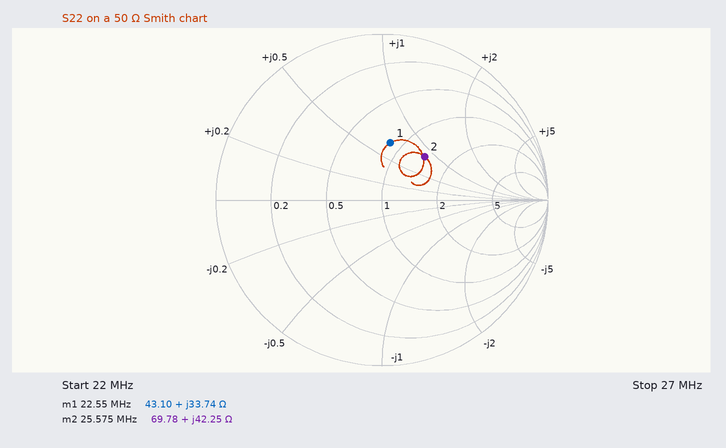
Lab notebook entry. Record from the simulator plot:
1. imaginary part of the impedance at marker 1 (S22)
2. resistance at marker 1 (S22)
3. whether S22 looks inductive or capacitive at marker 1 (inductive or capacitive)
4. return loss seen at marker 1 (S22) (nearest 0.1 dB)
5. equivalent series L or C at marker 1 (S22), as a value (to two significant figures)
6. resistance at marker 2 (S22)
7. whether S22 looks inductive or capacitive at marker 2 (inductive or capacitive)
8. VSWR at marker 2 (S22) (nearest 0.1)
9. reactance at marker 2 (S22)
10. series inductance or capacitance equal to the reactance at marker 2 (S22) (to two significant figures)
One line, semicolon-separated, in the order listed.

+33.74 Ω; 43.10 Ω; inductive; 9.2 dB; 240 nH; 69.78 Ω; inductive; 2.2; +42.25 Ω; 260 nH
